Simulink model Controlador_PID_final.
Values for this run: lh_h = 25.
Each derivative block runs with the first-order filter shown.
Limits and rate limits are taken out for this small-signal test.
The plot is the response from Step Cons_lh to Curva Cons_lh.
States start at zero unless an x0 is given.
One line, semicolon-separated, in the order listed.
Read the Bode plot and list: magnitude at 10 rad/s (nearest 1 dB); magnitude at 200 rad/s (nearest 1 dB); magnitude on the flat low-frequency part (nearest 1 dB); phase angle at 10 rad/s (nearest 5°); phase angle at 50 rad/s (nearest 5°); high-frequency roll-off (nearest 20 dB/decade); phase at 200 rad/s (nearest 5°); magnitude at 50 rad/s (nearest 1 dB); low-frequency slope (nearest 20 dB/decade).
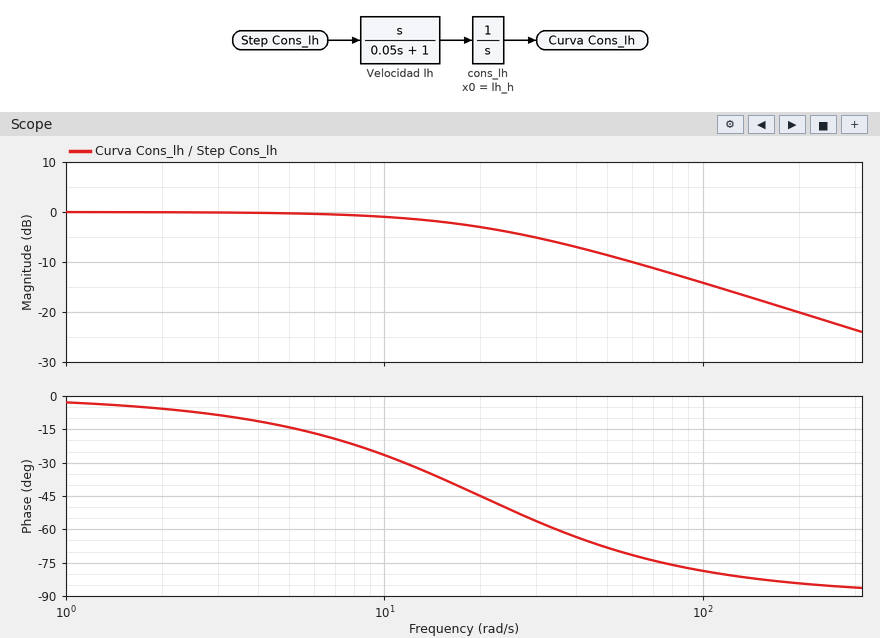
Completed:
-1 dB; -20 dB; 0 dB; -25°; -70°; -20 dB/decade; -85°; -9 dB; 0 dB/decade
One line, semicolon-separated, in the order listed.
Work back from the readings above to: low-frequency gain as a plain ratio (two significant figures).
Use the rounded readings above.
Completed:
1.0
